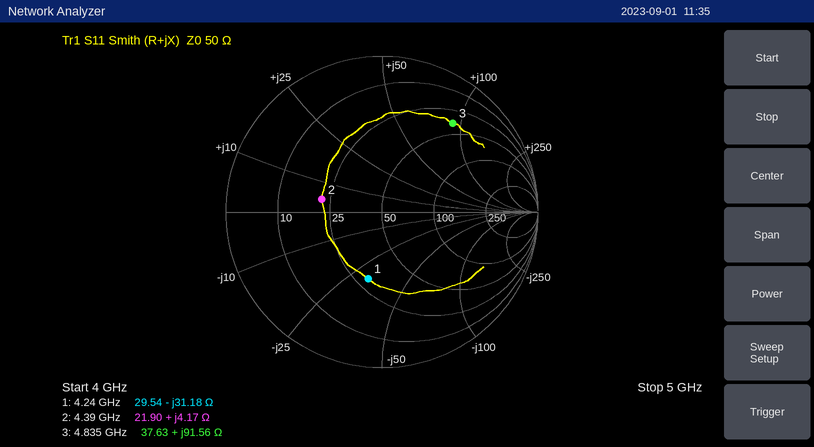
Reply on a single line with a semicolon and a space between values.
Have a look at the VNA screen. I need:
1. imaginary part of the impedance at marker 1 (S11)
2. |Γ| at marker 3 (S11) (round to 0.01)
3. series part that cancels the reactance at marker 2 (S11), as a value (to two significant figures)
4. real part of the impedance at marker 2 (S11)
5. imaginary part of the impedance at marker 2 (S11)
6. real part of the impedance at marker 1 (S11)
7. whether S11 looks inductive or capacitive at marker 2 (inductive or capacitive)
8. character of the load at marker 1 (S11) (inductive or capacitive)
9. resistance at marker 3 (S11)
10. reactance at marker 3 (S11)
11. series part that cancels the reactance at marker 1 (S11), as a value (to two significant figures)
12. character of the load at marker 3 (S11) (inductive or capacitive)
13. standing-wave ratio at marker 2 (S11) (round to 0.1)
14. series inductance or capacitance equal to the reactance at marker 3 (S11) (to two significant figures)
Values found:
-31.18 Ω; 0.73; 8.7 pF; 21.90 Ω; +4.17 Ω; 29.54 Ω; inductive; capacitive; 37.63 Ω; +91.56 Ω; 1.2 nH; inductive; 2.3; 3.0 nH
